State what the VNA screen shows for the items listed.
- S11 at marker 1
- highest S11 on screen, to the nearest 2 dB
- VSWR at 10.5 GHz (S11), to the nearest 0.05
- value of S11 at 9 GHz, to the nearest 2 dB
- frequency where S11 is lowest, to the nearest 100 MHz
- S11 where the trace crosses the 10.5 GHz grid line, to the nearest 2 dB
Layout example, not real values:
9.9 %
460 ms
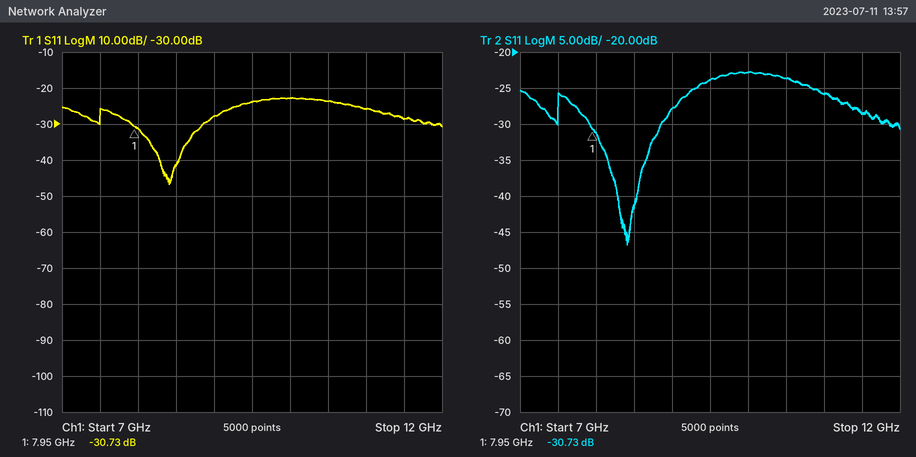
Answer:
-30.73 dB
-22 dB
1.15
-28 dB
8.4 GHz
-24 dB
